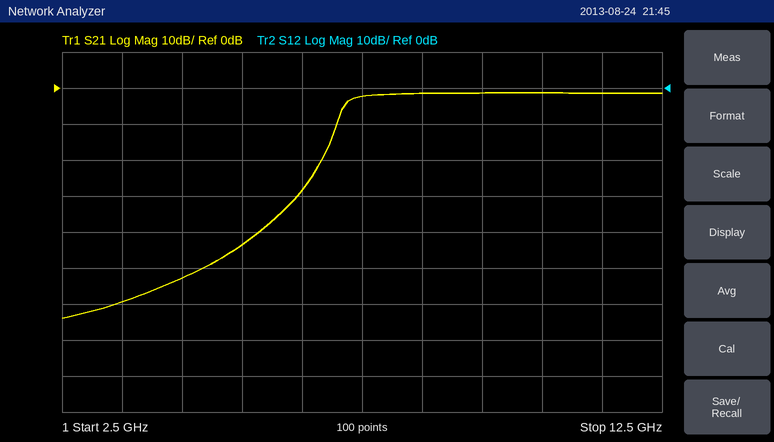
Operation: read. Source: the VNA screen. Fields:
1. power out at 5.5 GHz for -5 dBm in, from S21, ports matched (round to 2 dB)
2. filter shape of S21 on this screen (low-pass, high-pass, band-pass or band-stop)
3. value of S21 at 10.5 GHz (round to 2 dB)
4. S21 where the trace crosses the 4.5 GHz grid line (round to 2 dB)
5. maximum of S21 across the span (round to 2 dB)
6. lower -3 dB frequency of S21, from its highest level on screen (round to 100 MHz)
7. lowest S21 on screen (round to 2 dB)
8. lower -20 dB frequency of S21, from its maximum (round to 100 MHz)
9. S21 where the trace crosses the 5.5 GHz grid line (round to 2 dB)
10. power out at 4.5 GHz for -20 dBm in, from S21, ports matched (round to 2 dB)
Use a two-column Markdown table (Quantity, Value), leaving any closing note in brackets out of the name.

| Quantity | Value |
|---|---|
| power out at 5.5 GHz for -5 dBm in, from S21, ports matched | -48 dBm |
| filter shape of S21 on this screen | high-pass |
| value of S21 at 10.5 GHz | -2 dB |
| S21 where the trace crosses the 4.5 GHz grid line | -52 dB |
| maximum of S21 across the span | -2 dB |
| lower -3 dB frequency of S21, from its highest level on screen | 7.2 GHz |
| lowest S21 on screen | -64 dB |
| lower -20 dB frequency of S21, from its maximum | 6.8 GHz |
| S21 where the trace crosses the 5.5 GHz grid line | -44 dB |
| power out at 4.5 GHz for -20 dBm in, from S21, ports matched | -72 dBm |
